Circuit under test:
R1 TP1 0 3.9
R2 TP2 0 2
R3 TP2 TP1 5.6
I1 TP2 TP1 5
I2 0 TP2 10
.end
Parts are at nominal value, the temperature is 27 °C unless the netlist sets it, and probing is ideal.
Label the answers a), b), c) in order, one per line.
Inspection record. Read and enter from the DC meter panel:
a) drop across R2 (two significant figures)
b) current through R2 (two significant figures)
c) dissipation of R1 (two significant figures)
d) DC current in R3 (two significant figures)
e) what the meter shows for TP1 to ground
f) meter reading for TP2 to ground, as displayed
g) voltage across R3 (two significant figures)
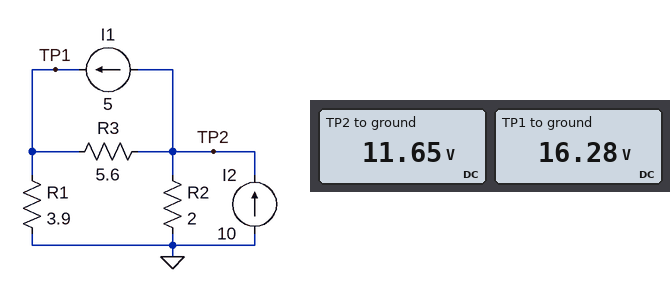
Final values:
a) 12 V
b) 5.8 A
c) 68 W
d) 830 mA
e) 16.28 V
f) 11.65 V
g) 4.6 V
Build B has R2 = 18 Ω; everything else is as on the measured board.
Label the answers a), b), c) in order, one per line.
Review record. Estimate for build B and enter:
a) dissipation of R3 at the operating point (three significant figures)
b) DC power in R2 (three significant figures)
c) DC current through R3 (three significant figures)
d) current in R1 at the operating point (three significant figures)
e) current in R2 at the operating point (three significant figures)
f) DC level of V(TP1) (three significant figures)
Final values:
a) 36.8 W
b) 107 W
c) 2.56 A
d) 7.56 A
e) 2.44 A
f) 29.5 V
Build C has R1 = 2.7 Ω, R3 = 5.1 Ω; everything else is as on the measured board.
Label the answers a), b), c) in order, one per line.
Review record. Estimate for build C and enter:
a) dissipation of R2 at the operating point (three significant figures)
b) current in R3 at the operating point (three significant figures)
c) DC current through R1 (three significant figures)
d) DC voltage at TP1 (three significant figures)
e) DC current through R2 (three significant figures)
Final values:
a) 57.4 W
b) 357 mA
c) 4.64 A
d) 12.5 V
e) 5.36 A
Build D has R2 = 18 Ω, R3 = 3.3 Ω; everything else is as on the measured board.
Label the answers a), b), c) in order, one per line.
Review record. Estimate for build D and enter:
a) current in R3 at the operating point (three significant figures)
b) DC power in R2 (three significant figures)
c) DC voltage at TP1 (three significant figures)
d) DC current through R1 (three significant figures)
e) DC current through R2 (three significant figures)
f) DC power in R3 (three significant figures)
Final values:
a) 2.80 A
b) 87.3 W
c) 30.4 V
d) 7.80 A
e) 2.20 A
f) 25.8 W
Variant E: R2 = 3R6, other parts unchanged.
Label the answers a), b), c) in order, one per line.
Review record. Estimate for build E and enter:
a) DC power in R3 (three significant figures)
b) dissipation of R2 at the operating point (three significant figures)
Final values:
a) 73.4 mW
b) 94.2 W
